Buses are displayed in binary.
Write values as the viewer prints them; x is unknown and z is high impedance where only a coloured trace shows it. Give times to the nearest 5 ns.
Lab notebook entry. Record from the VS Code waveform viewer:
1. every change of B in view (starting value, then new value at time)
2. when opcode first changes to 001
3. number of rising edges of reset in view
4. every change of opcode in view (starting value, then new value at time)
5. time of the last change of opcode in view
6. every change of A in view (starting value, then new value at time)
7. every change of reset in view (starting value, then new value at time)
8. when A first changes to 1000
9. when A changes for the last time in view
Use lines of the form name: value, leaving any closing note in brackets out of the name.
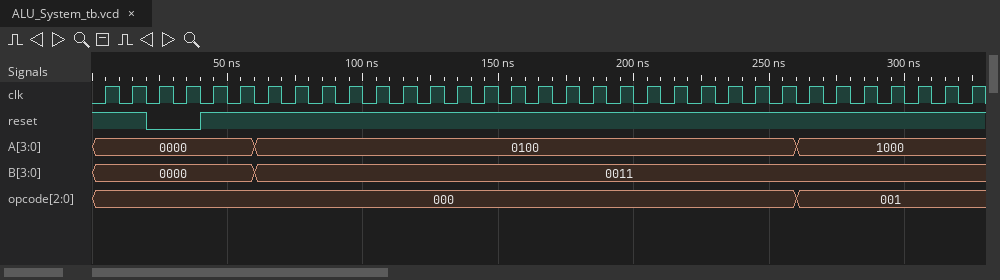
every change of B in view: 0000, 0011 at 60 ns
when opcode first changes to 001: 260 ns
number of rising edges of reset in view: 1
every change of opcode in view: 000, 001 at 260 ns
time of the last change of opcode in view: 260 ns
every change of A in view: 0000, 0100 at 60 ns, 1000 at 260 ns
every change of reset in view: 1, 0 at 20 ns, 1 at 40 ns
when A first changes to 1000: 260 ns
when A changes for the last time in view: 260 ns
